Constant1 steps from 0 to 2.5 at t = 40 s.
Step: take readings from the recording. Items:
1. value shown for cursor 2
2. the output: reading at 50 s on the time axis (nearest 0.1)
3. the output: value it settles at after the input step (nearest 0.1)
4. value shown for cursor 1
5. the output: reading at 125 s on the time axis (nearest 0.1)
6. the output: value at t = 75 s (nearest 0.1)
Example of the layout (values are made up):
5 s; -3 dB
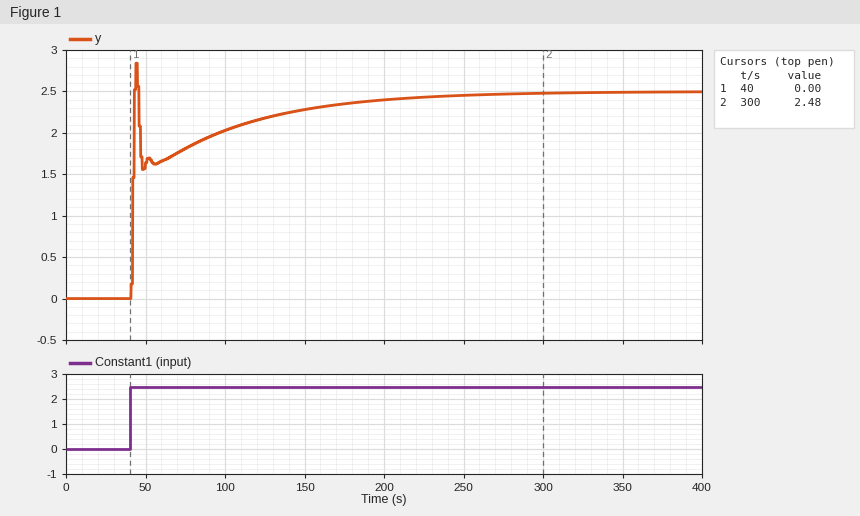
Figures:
2.48; 1.6; 2.5; 0.00; 2.2; 1.8
